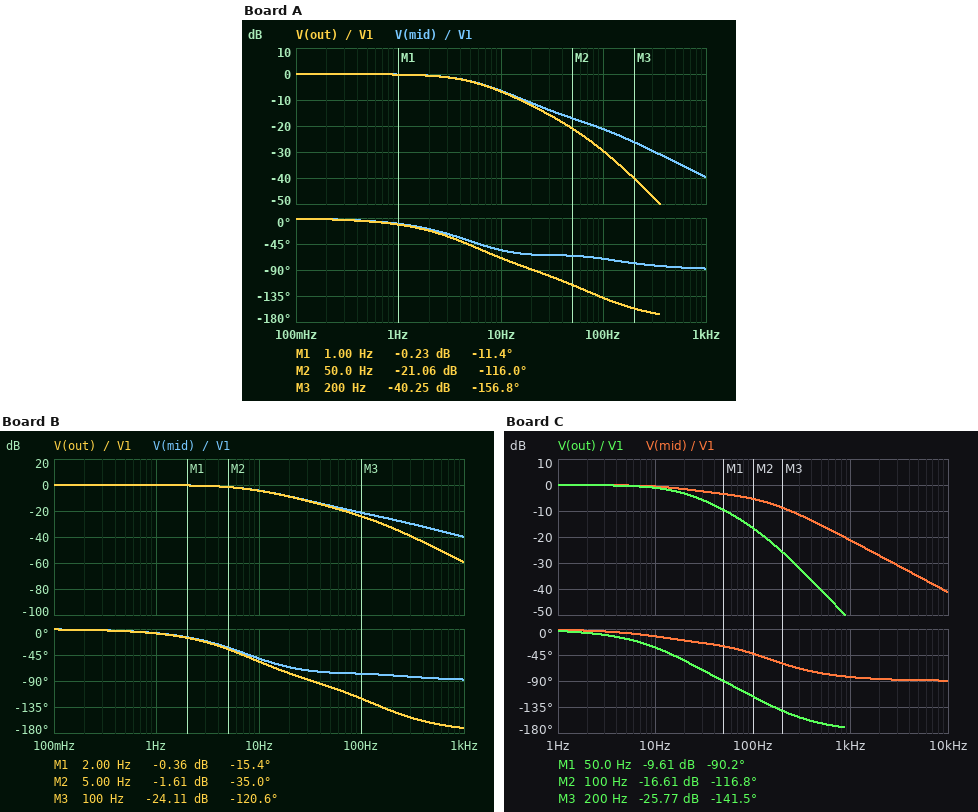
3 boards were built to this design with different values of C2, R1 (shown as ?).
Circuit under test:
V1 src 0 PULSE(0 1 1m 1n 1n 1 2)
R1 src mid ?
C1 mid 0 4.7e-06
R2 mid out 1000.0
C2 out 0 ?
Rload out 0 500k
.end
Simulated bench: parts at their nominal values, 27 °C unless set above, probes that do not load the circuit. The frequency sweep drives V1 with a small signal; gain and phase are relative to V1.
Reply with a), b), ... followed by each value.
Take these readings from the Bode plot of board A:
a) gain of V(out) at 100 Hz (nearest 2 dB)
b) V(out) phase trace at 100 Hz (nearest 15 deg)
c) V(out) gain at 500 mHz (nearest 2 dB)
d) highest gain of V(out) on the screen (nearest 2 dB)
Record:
a) -30 dB
b) -135 deg
c) 0 dB
d) 0 dB
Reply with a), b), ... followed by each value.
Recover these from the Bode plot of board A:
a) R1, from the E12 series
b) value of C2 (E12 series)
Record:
a) 3.3 kΩ
b) 3.9 µF
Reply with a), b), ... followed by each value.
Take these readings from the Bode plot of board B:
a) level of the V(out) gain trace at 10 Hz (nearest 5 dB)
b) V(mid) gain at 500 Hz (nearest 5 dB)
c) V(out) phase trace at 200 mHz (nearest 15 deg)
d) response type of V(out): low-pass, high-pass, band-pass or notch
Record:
a) -5 dB
b) -35 dB
c) 0 deg
d) low-pass
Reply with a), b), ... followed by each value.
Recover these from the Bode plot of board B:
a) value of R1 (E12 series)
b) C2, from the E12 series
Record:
a) 3.3 kΩ
b) 1.5 µF
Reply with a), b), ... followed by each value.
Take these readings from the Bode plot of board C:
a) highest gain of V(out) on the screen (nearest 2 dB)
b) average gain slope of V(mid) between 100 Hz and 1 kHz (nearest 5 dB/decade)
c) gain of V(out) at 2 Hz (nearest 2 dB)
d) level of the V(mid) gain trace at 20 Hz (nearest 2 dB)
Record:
a) 0 dB
b) -15 dB/decade
c) 0 dB
d) -2 dB
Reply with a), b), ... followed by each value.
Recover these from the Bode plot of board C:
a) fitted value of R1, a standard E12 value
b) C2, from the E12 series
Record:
a) 390 Ω
b) 5.6 µF
